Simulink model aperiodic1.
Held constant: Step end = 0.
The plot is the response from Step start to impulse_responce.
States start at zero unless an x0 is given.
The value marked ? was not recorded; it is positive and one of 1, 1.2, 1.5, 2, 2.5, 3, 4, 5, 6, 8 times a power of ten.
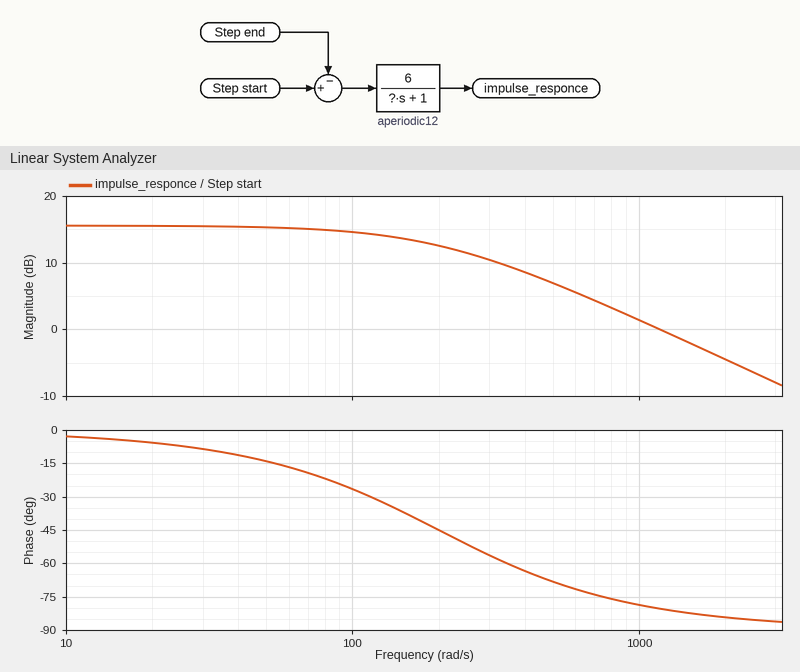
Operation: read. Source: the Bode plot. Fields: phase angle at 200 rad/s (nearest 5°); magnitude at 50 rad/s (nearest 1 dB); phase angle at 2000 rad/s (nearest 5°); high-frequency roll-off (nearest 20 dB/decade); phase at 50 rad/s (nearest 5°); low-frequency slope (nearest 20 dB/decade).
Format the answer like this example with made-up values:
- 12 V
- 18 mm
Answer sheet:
- -45°
- 15 dB
- -85°
- -20 dB/decade
- -15°
- 0 dB/decade
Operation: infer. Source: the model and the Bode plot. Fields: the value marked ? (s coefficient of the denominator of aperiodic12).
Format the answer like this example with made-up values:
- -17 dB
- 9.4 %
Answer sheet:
- 0.005
